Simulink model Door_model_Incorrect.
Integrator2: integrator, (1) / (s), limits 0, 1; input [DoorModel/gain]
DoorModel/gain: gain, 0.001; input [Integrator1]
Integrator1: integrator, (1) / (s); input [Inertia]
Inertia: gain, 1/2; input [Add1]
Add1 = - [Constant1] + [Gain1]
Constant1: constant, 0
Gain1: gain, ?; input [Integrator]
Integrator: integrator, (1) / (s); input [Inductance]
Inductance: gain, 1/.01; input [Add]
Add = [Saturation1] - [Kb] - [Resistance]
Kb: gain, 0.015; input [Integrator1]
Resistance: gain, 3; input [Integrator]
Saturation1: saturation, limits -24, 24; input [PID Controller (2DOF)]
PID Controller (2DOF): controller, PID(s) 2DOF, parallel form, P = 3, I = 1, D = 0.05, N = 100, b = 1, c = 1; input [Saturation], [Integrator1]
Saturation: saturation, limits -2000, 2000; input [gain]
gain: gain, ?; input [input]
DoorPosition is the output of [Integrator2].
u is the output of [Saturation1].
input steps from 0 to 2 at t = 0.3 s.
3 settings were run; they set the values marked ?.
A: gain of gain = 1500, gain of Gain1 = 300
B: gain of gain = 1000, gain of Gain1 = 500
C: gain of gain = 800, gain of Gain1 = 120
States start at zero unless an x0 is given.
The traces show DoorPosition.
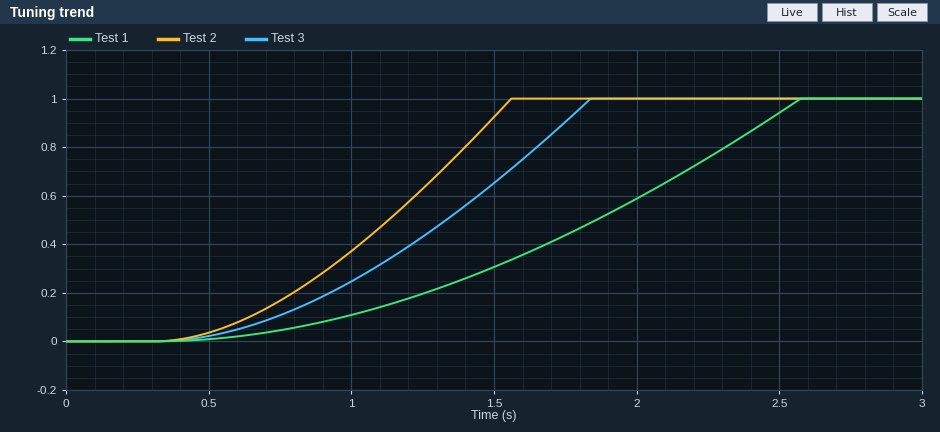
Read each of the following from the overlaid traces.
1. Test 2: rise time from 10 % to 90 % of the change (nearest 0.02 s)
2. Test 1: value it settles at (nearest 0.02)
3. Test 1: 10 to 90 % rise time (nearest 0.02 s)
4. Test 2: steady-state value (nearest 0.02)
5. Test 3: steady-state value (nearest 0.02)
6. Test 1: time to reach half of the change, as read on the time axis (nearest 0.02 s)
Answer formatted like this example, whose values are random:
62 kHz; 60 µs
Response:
0.84 s; 1.00; 1.48 s; 1.00; 1.00; 1.86 s
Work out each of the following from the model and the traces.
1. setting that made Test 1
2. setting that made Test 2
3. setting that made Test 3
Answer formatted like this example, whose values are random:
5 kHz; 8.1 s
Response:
C; B; A
